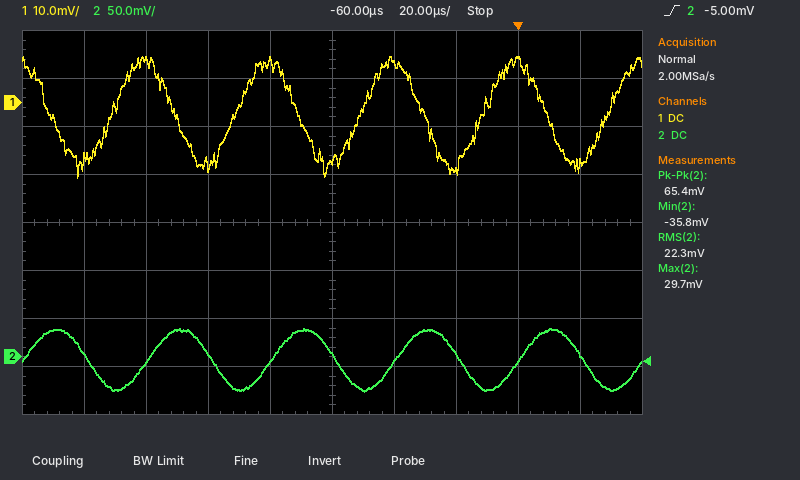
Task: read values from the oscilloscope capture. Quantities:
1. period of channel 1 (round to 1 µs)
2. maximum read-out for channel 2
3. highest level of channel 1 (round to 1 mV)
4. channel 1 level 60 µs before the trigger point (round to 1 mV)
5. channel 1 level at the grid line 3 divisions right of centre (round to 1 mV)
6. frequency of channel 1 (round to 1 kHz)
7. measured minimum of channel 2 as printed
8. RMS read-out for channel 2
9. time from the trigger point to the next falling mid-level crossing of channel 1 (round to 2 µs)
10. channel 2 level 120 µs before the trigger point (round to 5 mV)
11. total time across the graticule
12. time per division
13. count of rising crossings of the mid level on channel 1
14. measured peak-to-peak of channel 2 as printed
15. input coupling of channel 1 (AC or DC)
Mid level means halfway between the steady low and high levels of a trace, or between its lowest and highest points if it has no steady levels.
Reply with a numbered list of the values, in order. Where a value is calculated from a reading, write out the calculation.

1. 40 µs
2. 29.7 mV
3. 10 mV
4. -12 mV
5. 9 mV
6. 1 / 40 µs ≈ 25 kHz
7. -35.8 mV
8. 22.3 mV
9. 10 µs
10. -5 mV
11. 200 µs
12. 20 µs
13. 5
14. 65.4 mV
15. DC
